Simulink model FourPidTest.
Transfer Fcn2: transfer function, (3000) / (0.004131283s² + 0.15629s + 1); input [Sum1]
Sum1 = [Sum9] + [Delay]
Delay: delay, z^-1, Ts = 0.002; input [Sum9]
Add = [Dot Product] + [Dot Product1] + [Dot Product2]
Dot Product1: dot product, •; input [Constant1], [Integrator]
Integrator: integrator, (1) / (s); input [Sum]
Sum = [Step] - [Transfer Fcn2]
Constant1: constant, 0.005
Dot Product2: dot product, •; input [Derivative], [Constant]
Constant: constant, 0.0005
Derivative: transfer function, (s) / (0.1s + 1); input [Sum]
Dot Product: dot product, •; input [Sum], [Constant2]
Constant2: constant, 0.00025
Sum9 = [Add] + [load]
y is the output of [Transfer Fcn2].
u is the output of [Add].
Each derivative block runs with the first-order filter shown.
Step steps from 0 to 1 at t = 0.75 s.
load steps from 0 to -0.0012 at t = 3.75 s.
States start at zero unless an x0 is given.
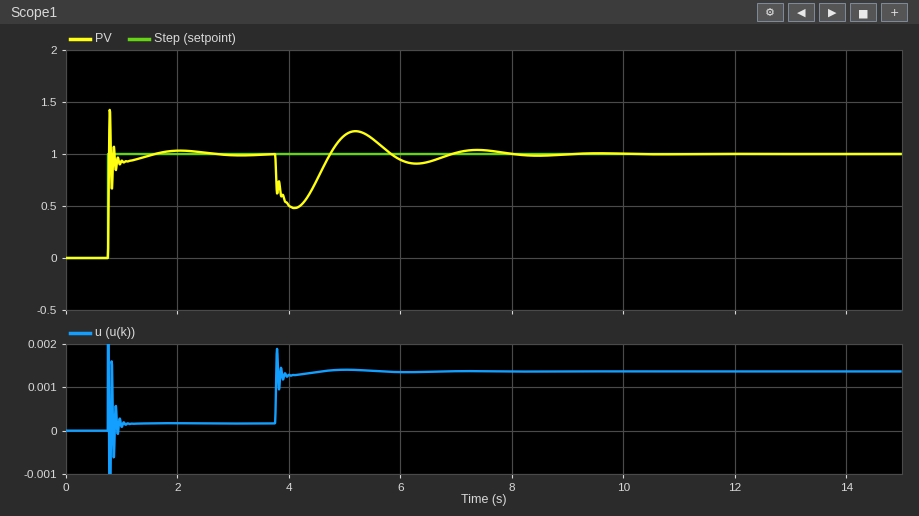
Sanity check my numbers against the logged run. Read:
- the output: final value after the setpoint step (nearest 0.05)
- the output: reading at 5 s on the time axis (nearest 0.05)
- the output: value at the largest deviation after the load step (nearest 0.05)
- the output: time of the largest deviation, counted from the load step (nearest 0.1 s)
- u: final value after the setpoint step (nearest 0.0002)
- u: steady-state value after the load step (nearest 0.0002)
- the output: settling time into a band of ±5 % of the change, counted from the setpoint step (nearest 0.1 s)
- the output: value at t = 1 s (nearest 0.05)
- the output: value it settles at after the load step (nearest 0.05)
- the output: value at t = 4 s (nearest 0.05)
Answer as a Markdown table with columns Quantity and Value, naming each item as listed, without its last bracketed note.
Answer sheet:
| Quantity | Value |
|---|---|
| the output: final value after the setpoint step | 1.00 |
| the output: reading at 5 s on the time axis | 1.20 |
| the output: value at the largest deviation after the load step | 0.50 |
| the output: time of the largest deviation, counted from the load step | 0.3 s |
| u: final value after the setpoint step | 0.0002 |
| u: steady-state value after the load step | 0.0014 |
| the output: settling time into a band of ±5 % of the change, counted from the setpoint step | 0.5 s |
| the output: value at t = 1 s | 0.95 |
| the output: value it settles at after the load step | 1.00 |
| the output: value at t = 4 s | 0.50 |
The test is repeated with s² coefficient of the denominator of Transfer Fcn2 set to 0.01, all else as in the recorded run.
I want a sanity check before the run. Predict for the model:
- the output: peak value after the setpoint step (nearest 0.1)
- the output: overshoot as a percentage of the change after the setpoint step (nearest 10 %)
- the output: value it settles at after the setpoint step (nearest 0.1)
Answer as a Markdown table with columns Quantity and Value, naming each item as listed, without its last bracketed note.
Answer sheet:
| Quantity | Value |
|---|---|
| the output: peak value after the setpoint step | 1.5 |
| the output: overshoot as a percentage of the change after the setpoint step | 50 % |
| the output: value it settles at after the setpoint step | 1.0 |
